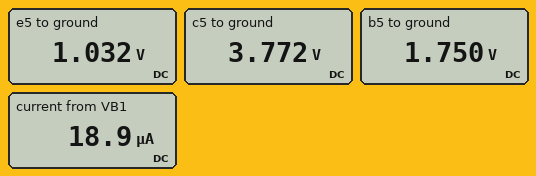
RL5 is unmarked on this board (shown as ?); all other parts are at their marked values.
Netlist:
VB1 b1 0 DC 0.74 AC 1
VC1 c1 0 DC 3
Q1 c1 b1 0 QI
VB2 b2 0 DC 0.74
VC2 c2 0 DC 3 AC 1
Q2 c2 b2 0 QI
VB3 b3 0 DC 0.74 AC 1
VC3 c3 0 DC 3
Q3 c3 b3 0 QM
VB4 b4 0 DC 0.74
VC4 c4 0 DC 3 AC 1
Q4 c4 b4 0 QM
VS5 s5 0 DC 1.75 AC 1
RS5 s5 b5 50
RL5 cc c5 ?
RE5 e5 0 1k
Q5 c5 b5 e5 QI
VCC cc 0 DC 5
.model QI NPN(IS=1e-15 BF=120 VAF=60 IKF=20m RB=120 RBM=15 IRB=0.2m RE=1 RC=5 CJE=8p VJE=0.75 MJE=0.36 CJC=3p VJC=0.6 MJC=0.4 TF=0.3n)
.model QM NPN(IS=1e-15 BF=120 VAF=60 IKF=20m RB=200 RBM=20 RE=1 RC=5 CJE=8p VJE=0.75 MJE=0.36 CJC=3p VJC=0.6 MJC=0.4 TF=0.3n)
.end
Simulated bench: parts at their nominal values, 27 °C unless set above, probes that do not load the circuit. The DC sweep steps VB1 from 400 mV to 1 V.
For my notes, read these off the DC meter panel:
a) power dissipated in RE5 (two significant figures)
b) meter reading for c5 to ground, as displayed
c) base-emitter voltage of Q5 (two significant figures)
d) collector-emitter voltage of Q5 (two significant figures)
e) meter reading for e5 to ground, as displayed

1.1 mW
3.772 V
720 mV
2.7 V
1.032 V
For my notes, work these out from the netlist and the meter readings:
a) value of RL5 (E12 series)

1.2 kΩ
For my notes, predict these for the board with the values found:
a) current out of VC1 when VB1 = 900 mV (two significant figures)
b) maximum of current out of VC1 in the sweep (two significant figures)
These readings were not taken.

34 mA
63 mA
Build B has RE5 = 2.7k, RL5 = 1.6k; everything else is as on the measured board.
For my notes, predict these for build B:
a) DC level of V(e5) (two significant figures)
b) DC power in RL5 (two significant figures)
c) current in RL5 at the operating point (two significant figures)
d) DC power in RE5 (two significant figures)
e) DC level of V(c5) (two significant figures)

1.1 V
240 µW
390 µA
420 µW
4.4 V
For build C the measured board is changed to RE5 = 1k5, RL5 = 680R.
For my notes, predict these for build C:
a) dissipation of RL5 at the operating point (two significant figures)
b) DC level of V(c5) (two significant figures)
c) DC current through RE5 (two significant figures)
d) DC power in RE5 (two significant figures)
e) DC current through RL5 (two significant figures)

320 µW
4.5 V
700 µA
730 µW
690 µA
